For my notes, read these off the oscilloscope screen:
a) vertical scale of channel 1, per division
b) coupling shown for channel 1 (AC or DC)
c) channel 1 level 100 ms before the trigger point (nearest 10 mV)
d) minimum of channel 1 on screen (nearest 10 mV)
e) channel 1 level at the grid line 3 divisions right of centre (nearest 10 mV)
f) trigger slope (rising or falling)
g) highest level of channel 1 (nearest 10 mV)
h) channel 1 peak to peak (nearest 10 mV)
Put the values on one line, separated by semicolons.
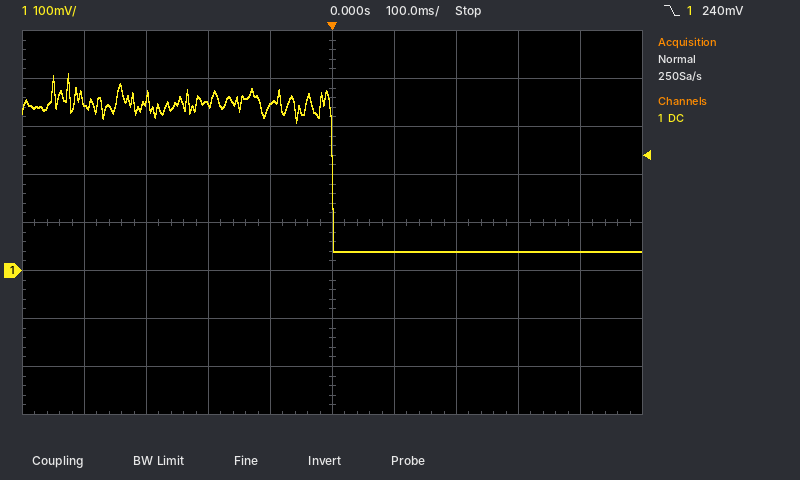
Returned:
100 mV; DC; 340 mV; 40 mV; 40 mV; falling; 410 mV; 370 mV
